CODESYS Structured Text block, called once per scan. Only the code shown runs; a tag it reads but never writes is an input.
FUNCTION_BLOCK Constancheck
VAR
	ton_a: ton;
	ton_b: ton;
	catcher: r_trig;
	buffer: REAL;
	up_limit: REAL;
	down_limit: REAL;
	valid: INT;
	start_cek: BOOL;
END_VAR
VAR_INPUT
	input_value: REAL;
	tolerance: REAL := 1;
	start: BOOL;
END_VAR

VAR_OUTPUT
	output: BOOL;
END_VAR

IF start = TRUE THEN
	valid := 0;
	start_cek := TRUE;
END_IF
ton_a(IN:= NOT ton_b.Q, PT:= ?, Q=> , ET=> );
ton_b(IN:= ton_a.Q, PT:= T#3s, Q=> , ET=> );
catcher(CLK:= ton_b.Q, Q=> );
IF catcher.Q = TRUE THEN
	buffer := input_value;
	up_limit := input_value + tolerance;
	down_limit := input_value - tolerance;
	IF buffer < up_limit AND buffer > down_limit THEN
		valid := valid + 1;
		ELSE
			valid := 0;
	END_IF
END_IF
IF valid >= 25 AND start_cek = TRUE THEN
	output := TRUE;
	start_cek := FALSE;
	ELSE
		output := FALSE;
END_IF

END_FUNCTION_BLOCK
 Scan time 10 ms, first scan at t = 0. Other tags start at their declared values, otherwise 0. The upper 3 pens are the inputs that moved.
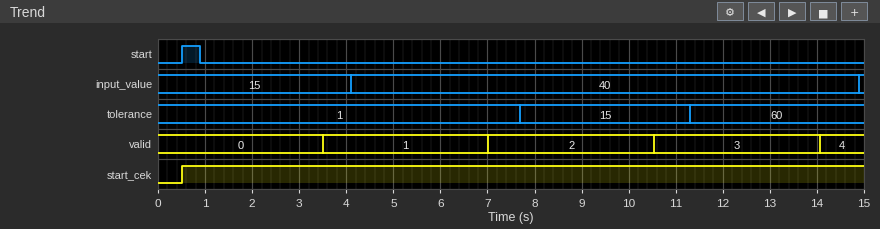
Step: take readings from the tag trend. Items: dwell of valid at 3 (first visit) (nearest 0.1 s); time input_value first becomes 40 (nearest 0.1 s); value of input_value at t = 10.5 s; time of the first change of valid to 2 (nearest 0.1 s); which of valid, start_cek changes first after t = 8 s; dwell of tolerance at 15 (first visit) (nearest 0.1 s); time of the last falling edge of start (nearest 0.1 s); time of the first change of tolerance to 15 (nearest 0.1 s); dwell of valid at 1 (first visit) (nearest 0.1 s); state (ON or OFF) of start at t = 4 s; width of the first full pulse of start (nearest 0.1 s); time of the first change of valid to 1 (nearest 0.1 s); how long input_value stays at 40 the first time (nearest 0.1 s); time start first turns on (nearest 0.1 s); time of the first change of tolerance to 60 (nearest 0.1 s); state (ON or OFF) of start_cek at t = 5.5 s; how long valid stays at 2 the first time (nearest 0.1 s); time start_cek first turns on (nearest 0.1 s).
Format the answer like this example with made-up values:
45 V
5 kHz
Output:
3.5 s
4.1 s
40
7.0 s
valid
3.6 s
0.9 s
7.7 s
3.5 s
OFF
0.4 s
3.5 s
10.8 s
0.5 s
11.3 s
ON
3.5 s
0.5 s
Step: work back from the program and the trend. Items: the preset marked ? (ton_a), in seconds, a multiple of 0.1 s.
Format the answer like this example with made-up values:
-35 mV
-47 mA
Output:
0.5 s
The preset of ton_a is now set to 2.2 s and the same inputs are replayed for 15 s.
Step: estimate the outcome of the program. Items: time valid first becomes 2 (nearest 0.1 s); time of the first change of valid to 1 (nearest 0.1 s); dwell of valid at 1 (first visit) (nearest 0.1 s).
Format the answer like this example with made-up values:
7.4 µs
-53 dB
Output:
10.4 s
5.2 s
5.2 s
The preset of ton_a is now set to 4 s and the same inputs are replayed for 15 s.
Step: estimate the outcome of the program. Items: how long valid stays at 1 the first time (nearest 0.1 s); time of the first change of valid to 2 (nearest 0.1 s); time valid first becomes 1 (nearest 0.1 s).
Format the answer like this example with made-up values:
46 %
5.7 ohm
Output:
7.0 s
14.0 s
7.0 s
